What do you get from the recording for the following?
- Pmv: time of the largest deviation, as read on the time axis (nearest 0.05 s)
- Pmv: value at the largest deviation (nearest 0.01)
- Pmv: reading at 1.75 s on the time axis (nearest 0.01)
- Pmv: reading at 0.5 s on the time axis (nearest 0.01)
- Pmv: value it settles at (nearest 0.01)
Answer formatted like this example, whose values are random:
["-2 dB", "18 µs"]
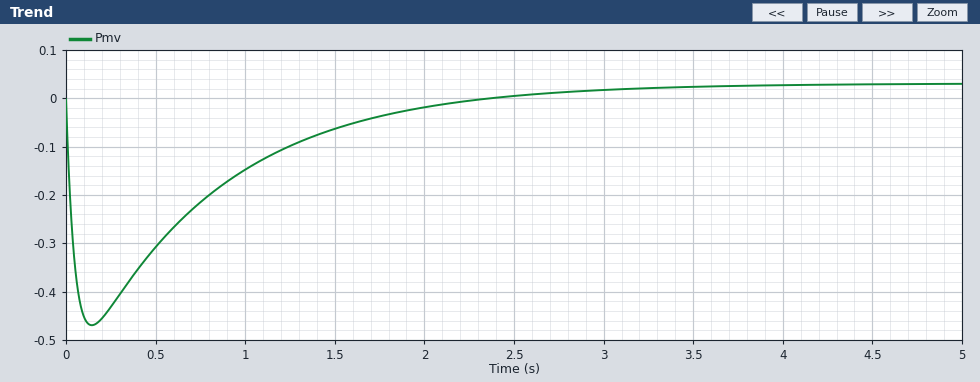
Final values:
["0.15 s", "-0.47", "-0.04", "-0.31", "0.03"]
